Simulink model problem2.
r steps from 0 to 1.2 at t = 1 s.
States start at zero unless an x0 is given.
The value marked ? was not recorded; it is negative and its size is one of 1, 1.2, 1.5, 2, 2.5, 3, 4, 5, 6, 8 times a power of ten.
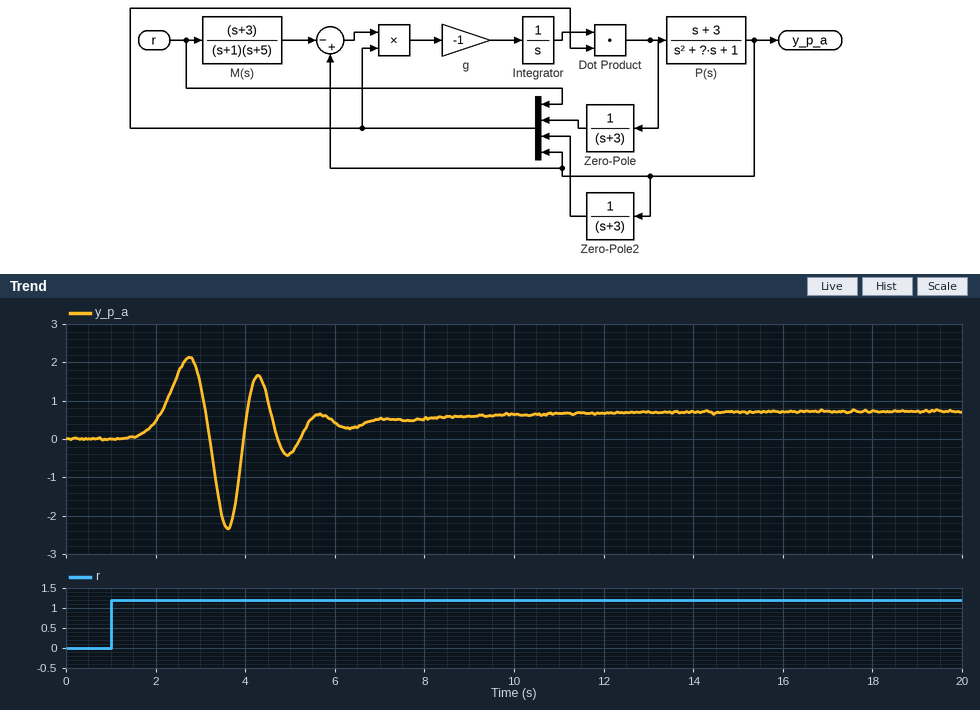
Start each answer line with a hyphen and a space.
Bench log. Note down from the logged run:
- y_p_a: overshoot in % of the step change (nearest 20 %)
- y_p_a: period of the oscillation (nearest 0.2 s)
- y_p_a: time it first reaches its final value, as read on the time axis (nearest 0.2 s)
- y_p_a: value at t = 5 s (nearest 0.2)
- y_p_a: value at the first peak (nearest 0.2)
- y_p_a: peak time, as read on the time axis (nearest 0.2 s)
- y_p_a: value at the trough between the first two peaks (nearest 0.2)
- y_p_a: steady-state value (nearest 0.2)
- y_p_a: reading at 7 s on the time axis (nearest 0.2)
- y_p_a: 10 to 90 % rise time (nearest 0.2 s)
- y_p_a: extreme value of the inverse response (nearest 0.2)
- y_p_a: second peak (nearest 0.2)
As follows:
- 200 %
- 1.6 s
- 2.2 s
- -0.4
- 2.2
- 2.8 s
- -2.4
- 0.8
- 0.6
- 0.6 s
- -2.4
- 1.6
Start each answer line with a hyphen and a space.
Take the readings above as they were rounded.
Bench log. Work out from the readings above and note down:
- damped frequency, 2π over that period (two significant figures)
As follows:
- 3.9 rad/s
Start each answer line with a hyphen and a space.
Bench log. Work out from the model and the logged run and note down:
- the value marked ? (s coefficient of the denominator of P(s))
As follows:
- -2
